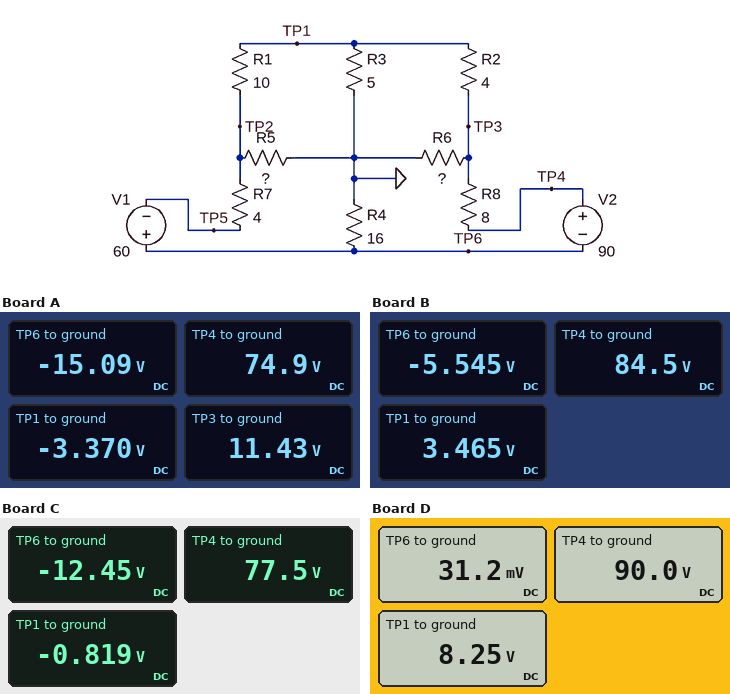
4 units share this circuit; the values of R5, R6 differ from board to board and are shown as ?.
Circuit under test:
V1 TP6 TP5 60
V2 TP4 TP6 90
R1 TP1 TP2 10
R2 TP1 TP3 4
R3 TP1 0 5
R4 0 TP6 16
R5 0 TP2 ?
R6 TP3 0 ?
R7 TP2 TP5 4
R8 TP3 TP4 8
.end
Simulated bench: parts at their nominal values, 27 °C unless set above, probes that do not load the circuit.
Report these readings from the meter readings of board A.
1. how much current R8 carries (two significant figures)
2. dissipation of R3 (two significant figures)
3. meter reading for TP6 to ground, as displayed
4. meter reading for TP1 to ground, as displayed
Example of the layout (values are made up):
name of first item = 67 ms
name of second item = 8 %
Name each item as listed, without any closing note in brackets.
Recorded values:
how much current R8 carries = 7.9 A
dissipation of R3 = 2.3 W
meter reading for TP6 to ground, as displayed = -15.09 V
meter reading for TP1 to ground, as displayed = -3.370 V
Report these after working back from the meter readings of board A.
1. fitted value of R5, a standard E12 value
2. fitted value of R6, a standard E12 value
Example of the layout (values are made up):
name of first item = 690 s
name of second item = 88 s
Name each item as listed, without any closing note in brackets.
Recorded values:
fitted value of R5, a standard E12 value = 18 Ω
fitted value of R6, a standard E12 value = 2.7 Ω
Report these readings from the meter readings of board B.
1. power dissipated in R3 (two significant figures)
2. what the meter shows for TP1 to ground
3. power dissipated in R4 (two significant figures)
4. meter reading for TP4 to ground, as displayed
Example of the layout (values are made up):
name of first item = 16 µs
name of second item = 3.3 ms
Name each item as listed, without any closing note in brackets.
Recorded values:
power dissipated in R3 = 2.4 W
what the meter shows for TP1 to ground = 3.465 V
power dissipated in R4 = 1.9 W
meter reading for TP4 to ground, as displayed = 84.5 V
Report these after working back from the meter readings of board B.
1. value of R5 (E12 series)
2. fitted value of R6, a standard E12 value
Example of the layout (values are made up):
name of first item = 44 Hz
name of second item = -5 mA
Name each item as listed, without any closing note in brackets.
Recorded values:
value of R5 = 10 Ω
fitted value of R6, a standard E12 value = 6.8 Ω
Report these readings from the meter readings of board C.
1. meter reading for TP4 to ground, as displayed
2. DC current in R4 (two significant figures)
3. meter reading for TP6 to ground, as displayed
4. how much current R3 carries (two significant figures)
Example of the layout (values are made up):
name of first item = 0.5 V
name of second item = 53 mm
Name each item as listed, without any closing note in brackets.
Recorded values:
meter reading for TP4 to ground, as displayed = 77.5 V
DC current in R4 = 780 mA
meter reading for TP6 to ground, as displayed = -12.45 V
how much current R3 carries = 160 mA
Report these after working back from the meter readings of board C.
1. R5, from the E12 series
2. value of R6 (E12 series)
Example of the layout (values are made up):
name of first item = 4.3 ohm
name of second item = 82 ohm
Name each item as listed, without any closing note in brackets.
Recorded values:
R5, from the E12 series = 18 Ω
value of R6 = 4.7 Ω
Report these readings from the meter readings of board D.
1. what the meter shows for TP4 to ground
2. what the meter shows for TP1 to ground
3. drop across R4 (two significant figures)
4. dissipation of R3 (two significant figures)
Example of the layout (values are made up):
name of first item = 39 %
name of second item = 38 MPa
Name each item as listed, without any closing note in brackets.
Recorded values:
what the meter shows for TP4 to ground = 90.0 V
what the meter shows for TP1 to ground = 8.25 V
drop across R4 = 31 mV
dissipation of R3 = 14 W
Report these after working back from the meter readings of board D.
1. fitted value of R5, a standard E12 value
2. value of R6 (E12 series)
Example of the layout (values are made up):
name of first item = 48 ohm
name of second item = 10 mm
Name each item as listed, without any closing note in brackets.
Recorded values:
fitted value of R5, a standard E12 value = 8.2 Ω
value of R6 = 15 Ω
